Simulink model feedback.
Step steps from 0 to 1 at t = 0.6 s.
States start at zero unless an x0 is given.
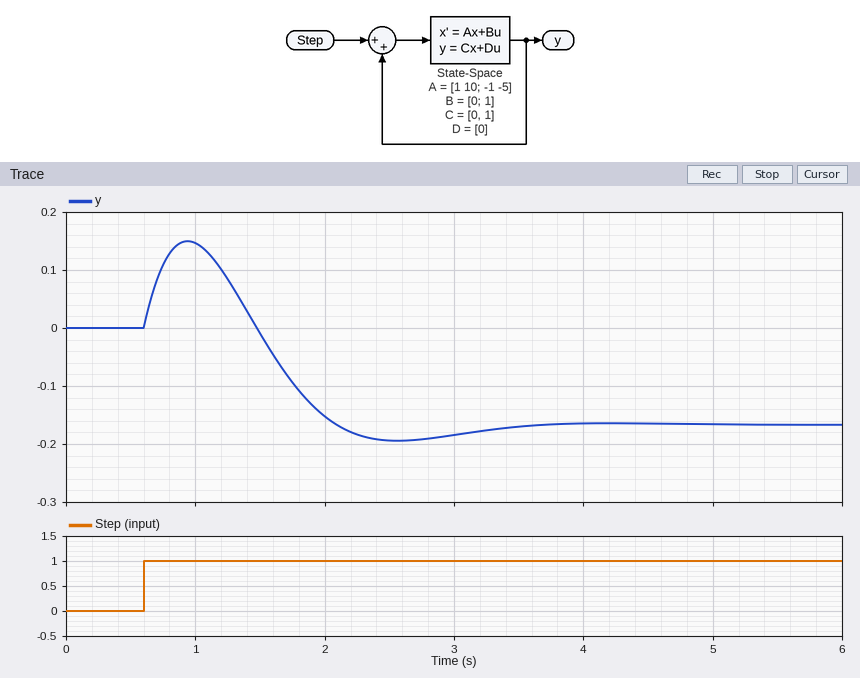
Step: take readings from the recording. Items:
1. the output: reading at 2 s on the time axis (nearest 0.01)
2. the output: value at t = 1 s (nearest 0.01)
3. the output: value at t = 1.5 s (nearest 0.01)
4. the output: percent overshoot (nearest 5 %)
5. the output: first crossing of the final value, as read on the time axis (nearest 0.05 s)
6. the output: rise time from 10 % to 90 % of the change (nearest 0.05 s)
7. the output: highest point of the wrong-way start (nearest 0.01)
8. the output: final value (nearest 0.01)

-0.15
0.15
-0.01
15 %
2.10 s
0.45 s
0.15
-0.17
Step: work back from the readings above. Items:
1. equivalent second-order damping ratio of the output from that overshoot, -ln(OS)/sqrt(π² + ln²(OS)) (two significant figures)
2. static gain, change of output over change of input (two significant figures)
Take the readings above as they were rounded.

0.52
-0.17
